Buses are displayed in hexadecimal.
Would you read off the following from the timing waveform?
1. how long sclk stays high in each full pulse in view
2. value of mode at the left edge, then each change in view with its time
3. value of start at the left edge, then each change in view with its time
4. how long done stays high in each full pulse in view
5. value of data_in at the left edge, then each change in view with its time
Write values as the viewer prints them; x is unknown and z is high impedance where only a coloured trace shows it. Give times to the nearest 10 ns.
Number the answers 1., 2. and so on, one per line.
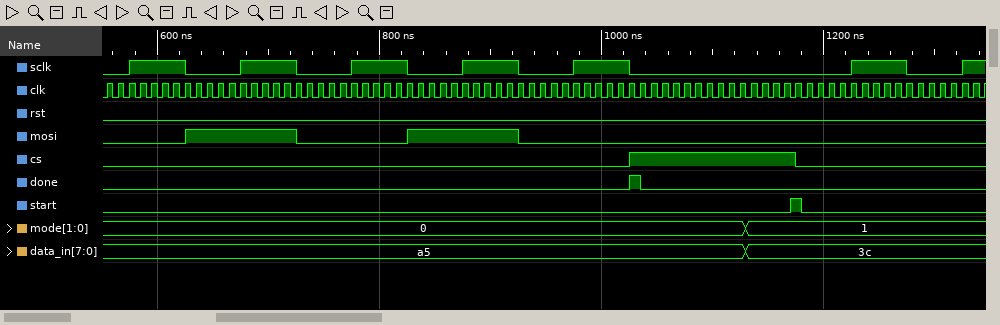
1. 50 ns, 50 ns, 50 ns, 50 ns, 50 ns, 50 ns
2. 0, 1 at 1130 ns
3. 0, 1 at 1170 ns, 0 at 1180 ns
4. 10 ns
5. a5, 3c at 1130 ns
